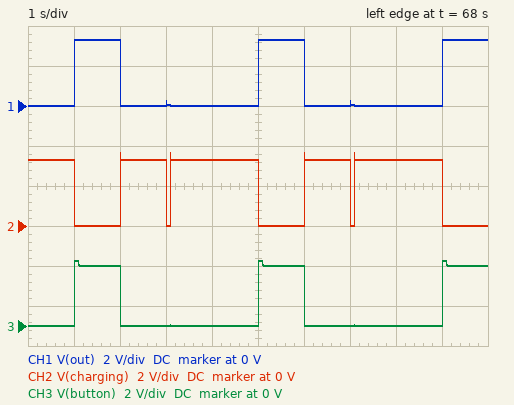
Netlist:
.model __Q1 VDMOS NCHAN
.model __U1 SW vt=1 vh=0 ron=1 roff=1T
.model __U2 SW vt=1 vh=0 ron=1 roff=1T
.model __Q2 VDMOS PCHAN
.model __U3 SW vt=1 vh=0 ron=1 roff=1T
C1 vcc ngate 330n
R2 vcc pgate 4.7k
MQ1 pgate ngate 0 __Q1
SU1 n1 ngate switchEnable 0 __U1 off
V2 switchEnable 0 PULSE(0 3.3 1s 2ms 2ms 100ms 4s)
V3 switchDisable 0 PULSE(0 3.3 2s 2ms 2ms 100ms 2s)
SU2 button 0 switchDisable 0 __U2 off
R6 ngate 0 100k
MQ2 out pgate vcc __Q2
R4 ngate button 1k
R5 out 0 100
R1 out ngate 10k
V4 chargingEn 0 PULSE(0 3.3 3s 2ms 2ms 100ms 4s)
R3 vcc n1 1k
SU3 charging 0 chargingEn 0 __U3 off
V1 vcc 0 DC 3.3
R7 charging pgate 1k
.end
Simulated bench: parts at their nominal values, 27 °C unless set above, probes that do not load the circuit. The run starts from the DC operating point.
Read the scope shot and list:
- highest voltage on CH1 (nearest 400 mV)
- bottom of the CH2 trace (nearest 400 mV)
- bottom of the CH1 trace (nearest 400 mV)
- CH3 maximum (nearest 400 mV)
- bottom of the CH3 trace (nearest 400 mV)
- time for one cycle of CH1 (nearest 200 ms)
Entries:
3.2 V
0 V
0 V
3.2 V
0 V
4.0 s
